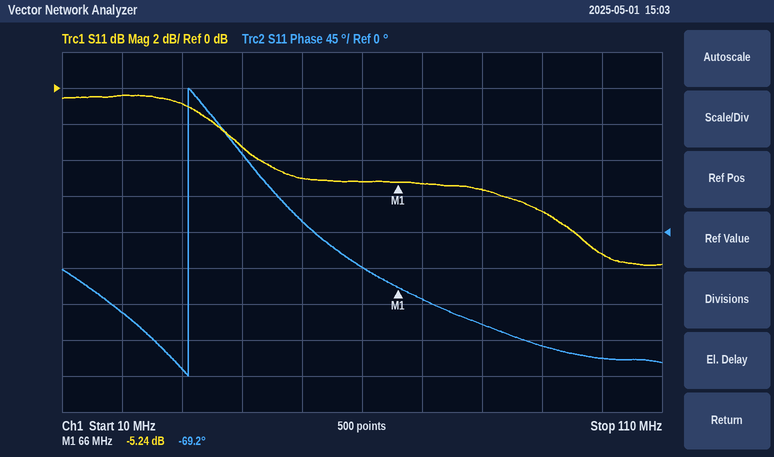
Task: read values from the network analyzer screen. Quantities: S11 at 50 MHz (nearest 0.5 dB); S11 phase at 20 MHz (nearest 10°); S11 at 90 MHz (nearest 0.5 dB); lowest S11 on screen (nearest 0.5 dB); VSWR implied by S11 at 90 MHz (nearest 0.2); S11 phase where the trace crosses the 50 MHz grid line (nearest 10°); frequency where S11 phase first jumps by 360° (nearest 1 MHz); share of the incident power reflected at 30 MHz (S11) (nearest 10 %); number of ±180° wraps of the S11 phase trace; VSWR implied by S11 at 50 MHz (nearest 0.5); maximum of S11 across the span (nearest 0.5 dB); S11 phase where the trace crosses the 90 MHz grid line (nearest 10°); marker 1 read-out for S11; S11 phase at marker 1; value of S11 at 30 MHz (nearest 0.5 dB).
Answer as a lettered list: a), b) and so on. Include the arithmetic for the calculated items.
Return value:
a) -5.0 dB
b) -100°
c) -7.0 dB
d) -10.0 dB
e) |Γ| = 10^(-7/20) = 0.4467; VSWR = (1 + 0.4467)/(1 − 0.4467) ≈ 2.6
f) 10°
g) 31 MHz
h) 10^(-1/10) ≈ 79.4 %, so 80 % to the nearest 10 %
i) 1
j) |Γ| = 10^(-5/20) = 0.5623; VSWR = (1 + 0.5623)/(1 − 0.5623) ≈ 3.57, so 3.5 to the nearest 0.5
k) -0.5 dB
l) -140°
m) -5.24 dB
n) -69.2°
o) -1.0 dB
